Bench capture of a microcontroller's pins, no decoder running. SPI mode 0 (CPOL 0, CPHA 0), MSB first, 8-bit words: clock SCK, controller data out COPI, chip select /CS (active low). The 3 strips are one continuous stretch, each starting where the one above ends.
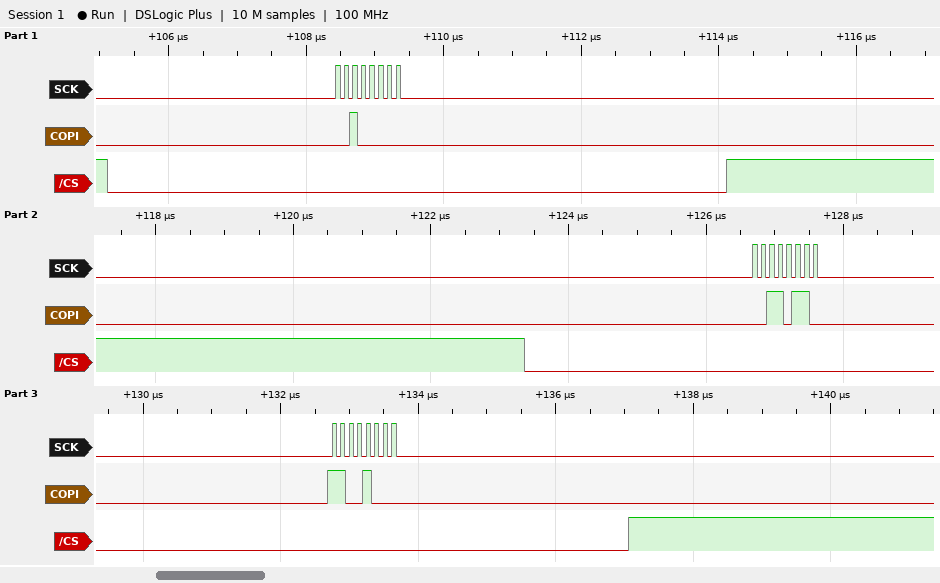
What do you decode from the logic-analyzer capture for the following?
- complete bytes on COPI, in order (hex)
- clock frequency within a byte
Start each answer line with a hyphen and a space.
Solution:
- 0x20 0x36 0xC8
- 8 MHz
